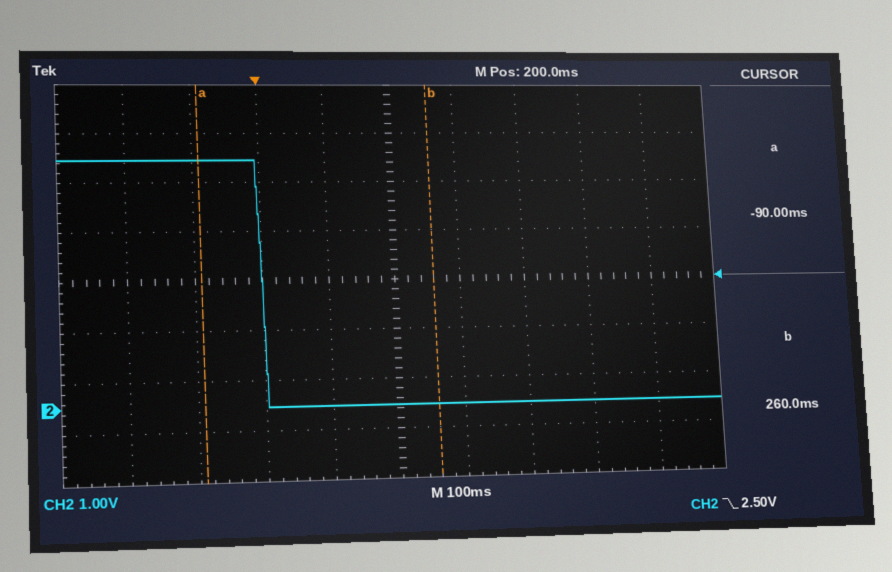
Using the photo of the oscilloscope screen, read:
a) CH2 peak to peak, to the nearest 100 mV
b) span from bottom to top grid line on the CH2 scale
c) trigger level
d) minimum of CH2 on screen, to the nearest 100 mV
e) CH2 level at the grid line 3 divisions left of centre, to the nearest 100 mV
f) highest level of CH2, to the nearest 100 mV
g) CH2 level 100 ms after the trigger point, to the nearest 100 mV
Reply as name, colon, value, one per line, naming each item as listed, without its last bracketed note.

CH2 peak to peak, to the nearest 100 mV: 5.0 V
span from bottom to top grid line on the CH2 scale: 8 V
trigger level: 2.50 V
minimum of CH2 on screen, to the nearest 100 mV: 0.0 V
CH2 level at the grid line 3 divisions left of centre, to the nearest 100 mV: 5.0 V
highest level of CH2, to the nearest 100 mV: 5.0 V
CH2 level 100 ms after the trigger point, to the nearest 100 mV: 0.0 V
